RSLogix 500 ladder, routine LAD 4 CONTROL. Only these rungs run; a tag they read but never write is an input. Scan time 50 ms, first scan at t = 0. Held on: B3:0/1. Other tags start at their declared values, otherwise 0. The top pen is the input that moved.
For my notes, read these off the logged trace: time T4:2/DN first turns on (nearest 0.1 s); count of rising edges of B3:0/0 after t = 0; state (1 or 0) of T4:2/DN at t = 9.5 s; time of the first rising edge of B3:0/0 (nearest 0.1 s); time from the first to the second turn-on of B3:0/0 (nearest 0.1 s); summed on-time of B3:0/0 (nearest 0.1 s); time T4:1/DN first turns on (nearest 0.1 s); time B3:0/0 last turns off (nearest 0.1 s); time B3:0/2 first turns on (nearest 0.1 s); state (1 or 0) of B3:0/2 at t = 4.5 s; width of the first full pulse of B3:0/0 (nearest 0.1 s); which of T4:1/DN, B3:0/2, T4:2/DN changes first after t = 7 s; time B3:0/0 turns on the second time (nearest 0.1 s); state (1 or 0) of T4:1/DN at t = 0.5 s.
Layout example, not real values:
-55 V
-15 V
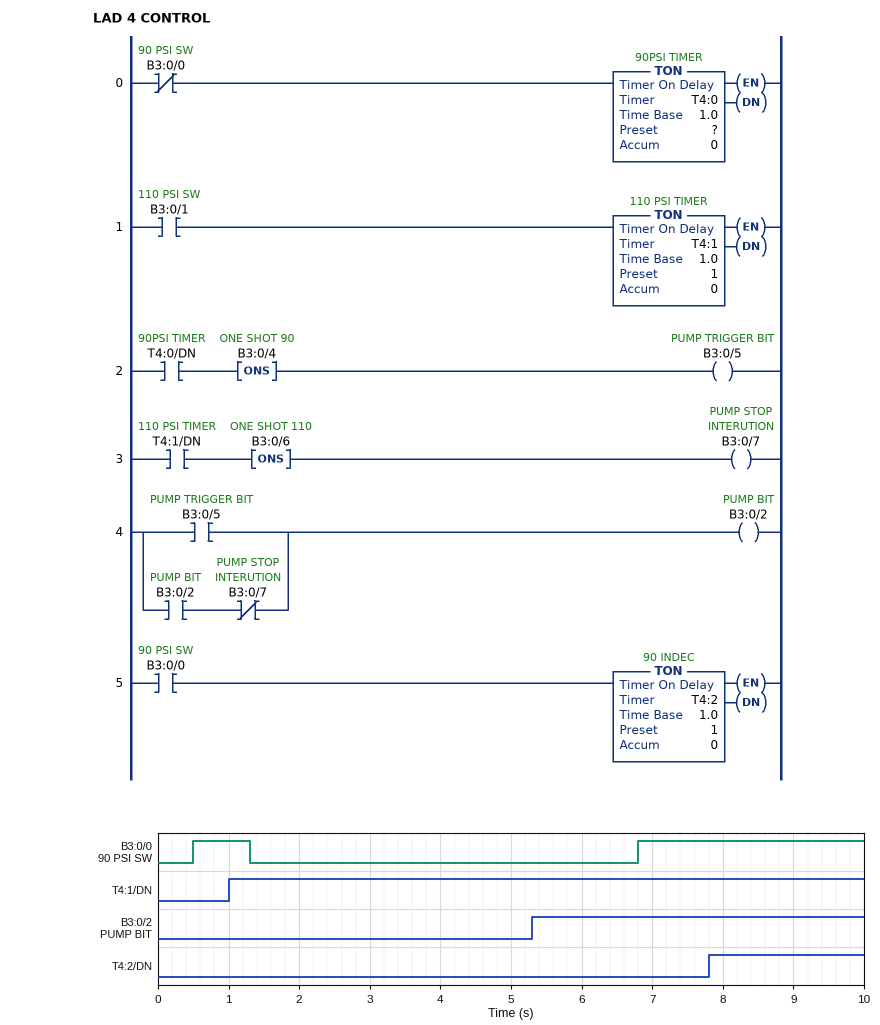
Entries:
7.8 s
2
1
0.5 s
6.3 s
4.0 s
1.0 s
1.3 s
5.3 s
0
0.8 s
T4:2/DN
6.8 s
0
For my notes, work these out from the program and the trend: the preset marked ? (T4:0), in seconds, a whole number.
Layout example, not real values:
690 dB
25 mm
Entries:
4 s
